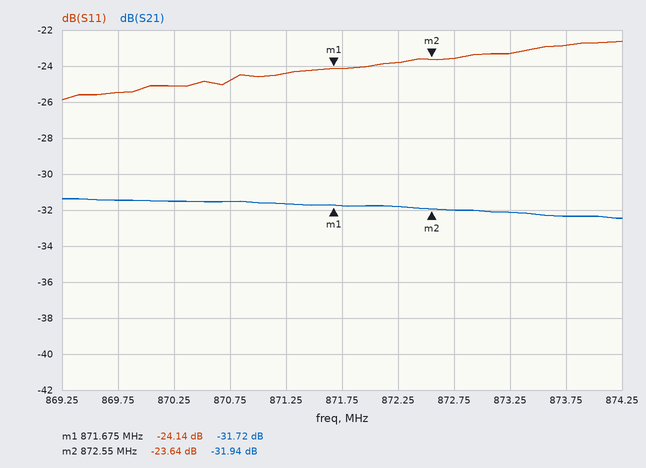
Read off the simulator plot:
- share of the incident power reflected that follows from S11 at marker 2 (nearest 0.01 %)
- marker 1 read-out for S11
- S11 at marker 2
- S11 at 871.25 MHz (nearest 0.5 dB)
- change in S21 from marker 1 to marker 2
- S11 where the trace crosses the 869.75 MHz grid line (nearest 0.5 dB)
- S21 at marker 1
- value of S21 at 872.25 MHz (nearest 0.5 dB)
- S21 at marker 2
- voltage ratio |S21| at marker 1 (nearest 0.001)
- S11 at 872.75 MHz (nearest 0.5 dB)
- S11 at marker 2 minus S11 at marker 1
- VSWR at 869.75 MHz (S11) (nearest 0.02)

0.43 %
-24.14 dB
-23.64 dB
-24.5 dB
-0.22 dB
-25.5 dB
-31.72 dB
-32.0 dB
-31.94 dB
0.026
-23.5 dB
0.50 dB
1.12
